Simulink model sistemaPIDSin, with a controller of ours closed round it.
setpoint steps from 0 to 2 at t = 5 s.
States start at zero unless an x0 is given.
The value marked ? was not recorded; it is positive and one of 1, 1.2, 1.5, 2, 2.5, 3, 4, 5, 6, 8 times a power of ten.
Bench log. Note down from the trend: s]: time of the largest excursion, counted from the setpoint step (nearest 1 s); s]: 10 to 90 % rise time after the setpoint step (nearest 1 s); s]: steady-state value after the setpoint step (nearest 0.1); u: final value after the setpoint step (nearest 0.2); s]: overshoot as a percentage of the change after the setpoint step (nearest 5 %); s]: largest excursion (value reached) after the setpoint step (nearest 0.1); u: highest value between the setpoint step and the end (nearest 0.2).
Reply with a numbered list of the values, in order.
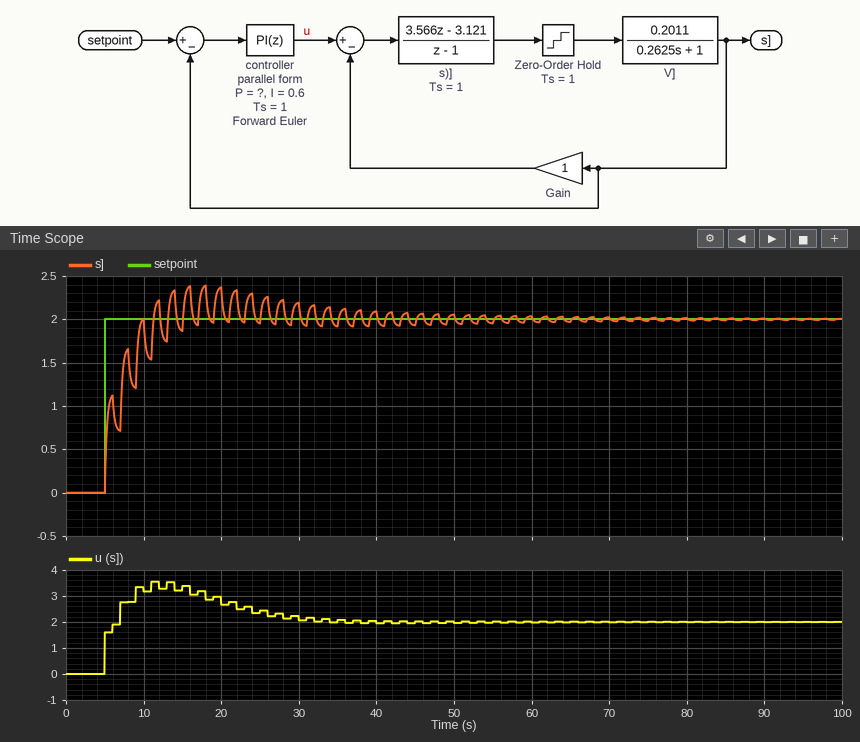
1. 13 s
2. 4 s
3. 2.0
4. 2.0
5. 20 %
6. 2.4
7. 3.6
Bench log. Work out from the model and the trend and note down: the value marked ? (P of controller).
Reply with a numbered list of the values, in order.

1. 0.8
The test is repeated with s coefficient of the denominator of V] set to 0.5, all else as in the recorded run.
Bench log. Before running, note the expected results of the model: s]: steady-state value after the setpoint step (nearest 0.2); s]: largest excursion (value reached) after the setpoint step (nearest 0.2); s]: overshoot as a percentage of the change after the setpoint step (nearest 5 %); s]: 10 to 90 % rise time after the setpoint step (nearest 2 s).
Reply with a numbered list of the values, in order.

1. 2.0
2. 2.2
3. 10 %
4. 6 s
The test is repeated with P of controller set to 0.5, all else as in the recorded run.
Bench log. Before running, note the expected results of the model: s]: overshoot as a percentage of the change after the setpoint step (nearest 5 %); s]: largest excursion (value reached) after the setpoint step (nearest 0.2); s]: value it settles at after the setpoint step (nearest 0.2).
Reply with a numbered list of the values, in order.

1. 10 %
2. 2.2
3. 2.0
